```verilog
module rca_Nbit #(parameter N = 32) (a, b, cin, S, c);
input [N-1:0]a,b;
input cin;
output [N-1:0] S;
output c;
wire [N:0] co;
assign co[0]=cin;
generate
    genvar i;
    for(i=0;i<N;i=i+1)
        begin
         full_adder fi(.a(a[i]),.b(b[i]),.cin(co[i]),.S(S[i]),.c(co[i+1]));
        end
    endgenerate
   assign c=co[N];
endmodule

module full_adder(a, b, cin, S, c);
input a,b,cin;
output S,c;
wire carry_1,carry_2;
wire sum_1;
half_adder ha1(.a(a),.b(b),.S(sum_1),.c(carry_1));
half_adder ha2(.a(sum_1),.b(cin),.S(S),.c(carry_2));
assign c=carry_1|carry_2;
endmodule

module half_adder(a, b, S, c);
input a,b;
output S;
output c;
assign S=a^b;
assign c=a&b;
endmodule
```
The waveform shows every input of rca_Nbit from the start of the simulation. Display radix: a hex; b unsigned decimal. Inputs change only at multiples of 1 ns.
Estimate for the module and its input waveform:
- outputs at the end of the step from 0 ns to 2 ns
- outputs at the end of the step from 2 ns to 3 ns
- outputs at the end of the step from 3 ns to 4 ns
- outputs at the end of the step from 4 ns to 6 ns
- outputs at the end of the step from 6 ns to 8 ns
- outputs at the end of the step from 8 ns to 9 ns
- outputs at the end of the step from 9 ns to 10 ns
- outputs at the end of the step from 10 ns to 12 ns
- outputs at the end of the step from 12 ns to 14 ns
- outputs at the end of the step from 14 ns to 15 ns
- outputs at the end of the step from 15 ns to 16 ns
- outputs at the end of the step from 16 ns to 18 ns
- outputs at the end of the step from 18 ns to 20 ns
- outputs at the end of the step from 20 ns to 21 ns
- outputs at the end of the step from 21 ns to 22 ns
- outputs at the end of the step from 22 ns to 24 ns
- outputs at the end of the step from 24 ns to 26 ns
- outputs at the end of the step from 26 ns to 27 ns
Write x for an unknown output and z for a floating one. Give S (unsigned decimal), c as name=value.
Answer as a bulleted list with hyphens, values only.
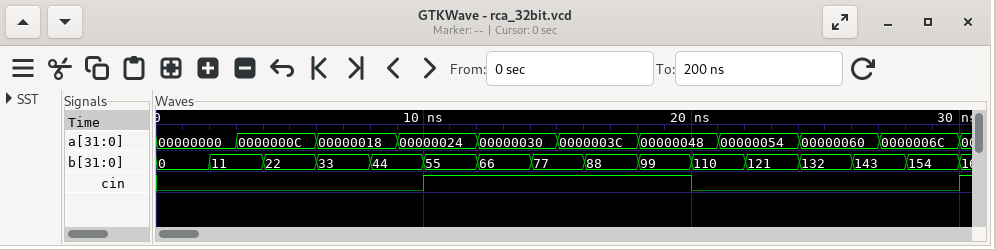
- S=0, c=0
- S=11, c=0
- S=23, c=0
- S=34, c=0
- S=57, c=0
- S=68, c=0
- S=80, c=0
- S=92, c=0
- S=115, c=0
- S=126, c=0
- S=138, c=0
- S=149, c=0
- S=172, c=0
- S=182, c=0
- S=194, c=0
- S=205, c=0
- S=228, c=0
- S=239, c=0
